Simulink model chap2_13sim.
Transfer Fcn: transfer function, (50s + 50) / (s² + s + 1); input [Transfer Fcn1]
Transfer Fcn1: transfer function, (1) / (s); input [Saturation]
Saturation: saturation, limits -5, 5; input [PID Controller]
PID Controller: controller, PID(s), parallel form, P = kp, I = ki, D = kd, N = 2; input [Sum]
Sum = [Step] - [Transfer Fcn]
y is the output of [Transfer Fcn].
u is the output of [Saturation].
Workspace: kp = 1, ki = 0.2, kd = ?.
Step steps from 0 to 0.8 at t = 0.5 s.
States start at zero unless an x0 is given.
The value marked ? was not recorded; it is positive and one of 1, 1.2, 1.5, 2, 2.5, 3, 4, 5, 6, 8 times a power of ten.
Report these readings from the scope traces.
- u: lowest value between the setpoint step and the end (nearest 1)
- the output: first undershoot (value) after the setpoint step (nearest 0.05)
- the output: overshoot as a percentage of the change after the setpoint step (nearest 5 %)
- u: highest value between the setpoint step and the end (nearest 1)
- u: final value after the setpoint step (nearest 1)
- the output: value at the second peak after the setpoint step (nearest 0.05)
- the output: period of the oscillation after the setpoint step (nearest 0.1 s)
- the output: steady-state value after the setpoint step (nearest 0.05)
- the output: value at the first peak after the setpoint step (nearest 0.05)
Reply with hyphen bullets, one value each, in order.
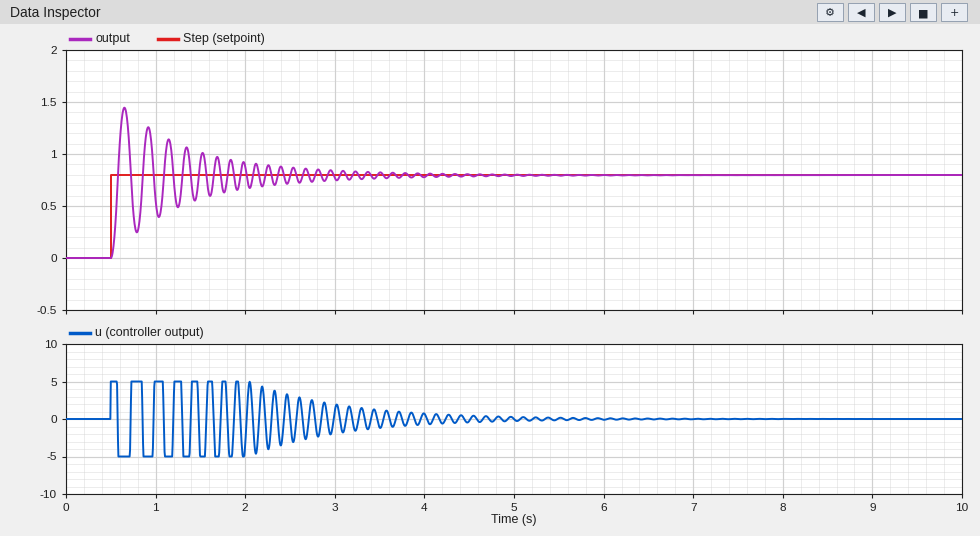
- -5
- 0.25
- 80 %
- 5
- 0
- 1.25
- 0.3 s
- 0.80
- 1.45
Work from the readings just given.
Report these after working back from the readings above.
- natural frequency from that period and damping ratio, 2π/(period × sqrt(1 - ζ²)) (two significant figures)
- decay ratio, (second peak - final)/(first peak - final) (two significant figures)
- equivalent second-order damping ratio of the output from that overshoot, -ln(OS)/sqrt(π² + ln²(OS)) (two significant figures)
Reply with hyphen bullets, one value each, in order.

- 21 rad/s
- 0.69
- 0.071
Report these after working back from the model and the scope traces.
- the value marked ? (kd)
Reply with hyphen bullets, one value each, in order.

- 20
